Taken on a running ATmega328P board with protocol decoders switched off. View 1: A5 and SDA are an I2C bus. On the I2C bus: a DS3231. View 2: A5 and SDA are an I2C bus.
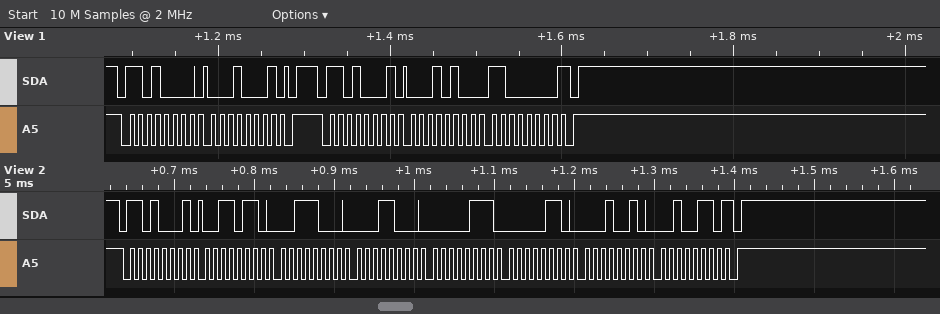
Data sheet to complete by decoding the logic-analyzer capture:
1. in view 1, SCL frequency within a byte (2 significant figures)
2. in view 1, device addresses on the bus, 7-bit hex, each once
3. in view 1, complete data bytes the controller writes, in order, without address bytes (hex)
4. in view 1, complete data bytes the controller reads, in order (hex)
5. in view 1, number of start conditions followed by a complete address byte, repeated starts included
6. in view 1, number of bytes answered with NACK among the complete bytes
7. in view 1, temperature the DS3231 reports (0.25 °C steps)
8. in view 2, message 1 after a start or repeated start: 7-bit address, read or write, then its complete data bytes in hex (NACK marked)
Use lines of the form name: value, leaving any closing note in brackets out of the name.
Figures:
in view 1, SCL frequency within a byte: 100 kHz
in view 1, device addresses on the bus, 7-bit hex, each once: 0x68
in view 1, complete data bytes the controller writes, in order, without address bytes: 11
in view 1, complete data bytes the controller reads, in order: 14 C0
in view 1, number of start conditions followed by a complete address byte, repeated starts included: 2
in view 1, number of bytes answered with NACK among the complete bytes: 1
in view 1, temperature the DS3231 reports: 20.75 °C
in view 2, message 1 after a start or repeated start: 7-bit address, read or write, then its complete data bytes in hex: 0x68 read: 36 38 18 07 06 12 26 NACK
